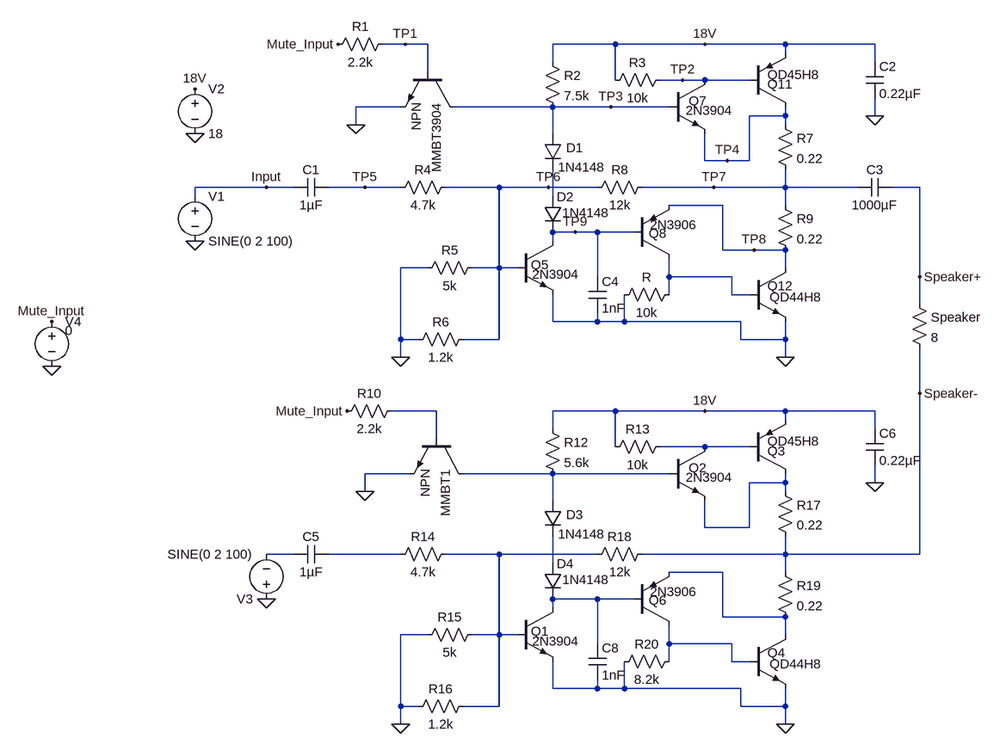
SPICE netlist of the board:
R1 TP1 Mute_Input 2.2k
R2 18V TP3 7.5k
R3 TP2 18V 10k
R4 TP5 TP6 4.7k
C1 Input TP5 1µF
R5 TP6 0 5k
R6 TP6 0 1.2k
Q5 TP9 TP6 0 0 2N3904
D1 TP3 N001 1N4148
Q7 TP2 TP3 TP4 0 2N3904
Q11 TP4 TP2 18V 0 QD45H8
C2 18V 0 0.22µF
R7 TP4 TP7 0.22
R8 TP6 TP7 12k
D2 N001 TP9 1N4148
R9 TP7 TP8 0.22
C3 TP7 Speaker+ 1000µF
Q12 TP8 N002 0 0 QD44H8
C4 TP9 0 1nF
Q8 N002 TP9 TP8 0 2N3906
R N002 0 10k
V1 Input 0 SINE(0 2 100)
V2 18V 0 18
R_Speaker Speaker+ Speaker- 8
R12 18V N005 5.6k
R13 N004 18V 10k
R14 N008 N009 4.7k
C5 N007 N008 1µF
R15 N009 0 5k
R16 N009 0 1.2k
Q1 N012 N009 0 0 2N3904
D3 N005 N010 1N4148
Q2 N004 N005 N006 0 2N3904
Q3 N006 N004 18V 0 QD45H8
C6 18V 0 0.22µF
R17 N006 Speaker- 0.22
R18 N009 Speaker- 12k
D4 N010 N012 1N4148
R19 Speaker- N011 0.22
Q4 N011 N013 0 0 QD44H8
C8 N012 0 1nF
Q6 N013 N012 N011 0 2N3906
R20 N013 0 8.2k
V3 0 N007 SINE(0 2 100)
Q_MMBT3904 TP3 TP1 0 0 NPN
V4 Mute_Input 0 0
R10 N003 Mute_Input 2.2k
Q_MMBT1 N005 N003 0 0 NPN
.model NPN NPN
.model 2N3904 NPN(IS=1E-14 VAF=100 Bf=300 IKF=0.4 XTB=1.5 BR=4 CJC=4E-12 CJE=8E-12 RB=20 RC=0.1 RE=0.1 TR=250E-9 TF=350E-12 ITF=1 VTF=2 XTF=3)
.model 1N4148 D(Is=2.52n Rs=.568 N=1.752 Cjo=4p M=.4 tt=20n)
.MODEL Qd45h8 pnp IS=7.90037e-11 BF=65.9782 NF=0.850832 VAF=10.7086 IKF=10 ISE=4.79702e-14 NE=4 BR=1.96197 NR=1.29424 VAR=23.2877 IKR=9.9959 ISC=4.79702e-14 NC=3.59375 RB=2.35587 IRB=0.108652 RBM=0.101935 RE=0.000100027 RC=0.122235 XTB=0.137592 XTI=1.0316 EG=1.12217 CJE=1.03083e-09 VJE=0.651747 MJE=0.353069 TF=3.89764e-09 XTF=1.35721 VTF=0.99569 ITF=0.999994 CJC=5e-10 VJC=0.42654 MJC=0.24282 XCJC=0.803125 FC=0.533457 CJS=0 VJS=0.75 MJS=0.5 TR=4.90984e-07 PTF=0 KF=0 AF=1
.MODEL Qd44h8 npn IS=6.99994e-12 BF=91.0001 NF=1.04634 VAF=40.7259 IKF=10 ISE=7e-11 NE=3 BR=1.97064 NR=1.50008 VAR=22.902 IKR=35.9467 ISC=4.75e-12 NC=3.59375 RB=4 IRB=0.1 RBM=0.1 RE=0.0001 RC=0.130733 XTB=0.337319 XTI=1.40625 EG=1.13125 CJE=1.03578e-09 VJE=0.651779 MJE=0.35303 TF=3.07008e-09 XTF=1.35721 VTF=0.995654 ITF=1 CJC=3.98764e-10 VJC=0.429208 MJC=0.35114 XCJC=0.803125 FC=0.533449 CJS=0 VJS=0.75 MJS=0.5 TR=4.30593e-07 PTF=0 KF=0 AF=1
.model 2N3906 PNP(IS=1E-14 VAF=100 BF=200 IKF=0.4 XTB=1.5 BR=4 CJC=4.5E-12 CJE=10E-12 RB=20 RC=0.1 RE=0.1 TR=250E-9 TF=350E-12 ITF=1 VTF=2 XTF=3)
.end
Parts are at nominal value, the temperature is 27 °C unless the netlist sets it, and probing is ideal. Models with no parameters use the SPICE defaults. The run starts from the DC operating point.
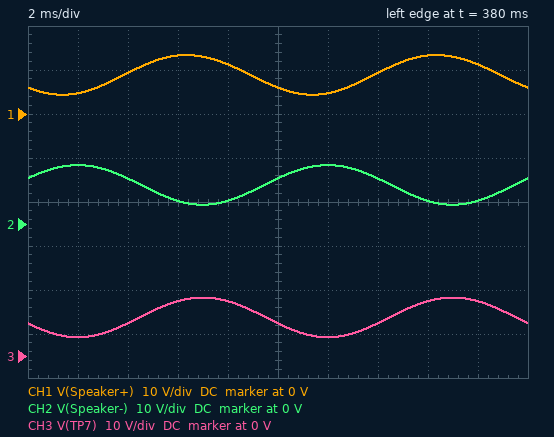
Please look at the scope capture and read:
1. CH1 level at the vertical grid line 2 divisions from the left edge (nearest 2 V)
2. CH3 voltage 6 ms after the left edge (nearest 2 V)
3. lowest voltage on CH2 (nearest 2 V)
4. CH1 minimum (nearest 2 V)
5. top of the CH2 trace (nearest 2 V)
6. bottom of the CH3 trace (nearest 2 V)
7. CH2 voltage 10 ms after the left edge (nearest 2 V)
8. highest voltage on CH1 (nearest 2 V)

10 V
12 V
4 V
4 V
14 V
4 V
10 V
14 V
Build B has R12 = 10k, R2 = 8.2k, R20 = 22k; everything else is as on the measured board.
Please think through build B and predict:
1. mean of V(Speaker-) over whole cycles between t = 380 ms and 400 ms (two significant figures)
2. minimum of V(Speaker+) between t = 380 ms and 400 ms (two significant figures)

8.7 V
4.2 V
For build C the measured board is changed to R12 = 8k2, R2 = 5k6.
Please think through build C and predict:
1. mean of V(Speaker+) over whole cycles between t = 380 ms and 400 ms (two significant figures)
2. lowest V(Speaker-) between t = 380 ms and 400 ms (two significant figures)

8.8 V
4.2 V
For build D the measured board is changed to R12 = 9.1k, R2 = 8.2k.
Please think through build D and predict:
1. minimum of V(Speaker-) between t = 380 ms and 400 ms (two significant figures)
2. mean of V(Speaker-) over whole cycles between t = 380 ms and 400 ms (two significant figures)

4.2 V
8.7 V
